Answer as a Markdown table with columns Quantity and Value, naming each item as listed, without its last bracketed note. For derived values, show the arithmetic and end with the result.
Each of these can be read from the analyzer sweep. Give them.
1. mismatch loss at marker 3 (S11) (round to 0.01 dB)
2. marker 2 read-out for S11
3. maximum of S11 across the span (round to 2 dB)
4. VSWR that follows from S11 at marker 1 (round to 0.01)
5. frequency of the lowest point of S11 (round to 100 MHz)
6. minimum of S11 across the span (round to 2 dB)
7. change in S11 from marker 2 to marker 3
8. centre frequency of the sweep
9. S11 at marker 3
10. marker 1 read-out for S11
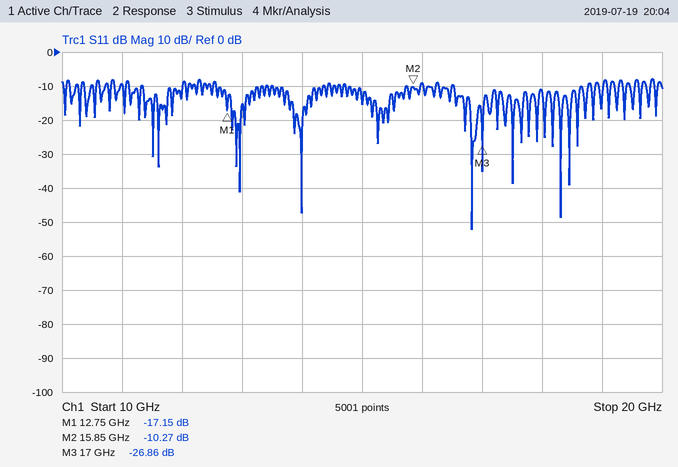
| Quantity | Value |
|---|---|
| mismatch loss at marker 3 (S11) | −10 log10(1 − 10^(-26.86/10)) ≈ 0.01 dB |
| marker 2 read-out for S11 | -10.27 dB |
| maximum of S11 across the span | -8 dB |
| VSWR that follows from S11 at marker 1 | (1 + 0.1388)/(1 − 0.1388) ≈ 1.32 |
| frequency of the lowest point of S11 | 16.8 GHz |
| minimum of S11 across the span | -52 dB |
| change in S11 from marker 2 to marker 3 | -26.86 − (-10.27) = -16.59 dB |
| centre frequency of the sweep | 15 GHz |
| S11 at marker 3 | -26.86 dB |
| marker 1 read-out for S11 | -17.15 dB |
